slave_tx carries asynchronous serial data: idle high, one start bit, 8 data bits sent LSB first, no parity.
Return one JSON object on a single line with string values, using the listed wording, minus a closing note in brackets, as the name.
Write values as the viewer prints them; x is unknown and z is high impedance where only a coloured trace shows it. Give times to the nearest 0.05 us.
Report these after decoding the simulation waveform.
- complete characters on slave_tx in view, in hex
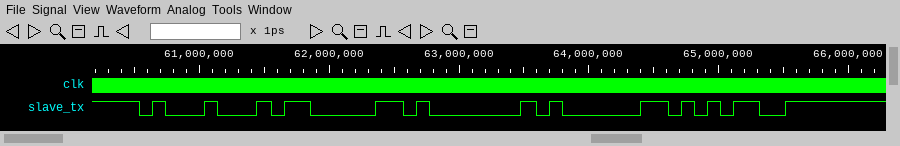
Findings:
{"complete characters on slave_tx in view, in hex": "11, 83, 01, 81, 35"}
